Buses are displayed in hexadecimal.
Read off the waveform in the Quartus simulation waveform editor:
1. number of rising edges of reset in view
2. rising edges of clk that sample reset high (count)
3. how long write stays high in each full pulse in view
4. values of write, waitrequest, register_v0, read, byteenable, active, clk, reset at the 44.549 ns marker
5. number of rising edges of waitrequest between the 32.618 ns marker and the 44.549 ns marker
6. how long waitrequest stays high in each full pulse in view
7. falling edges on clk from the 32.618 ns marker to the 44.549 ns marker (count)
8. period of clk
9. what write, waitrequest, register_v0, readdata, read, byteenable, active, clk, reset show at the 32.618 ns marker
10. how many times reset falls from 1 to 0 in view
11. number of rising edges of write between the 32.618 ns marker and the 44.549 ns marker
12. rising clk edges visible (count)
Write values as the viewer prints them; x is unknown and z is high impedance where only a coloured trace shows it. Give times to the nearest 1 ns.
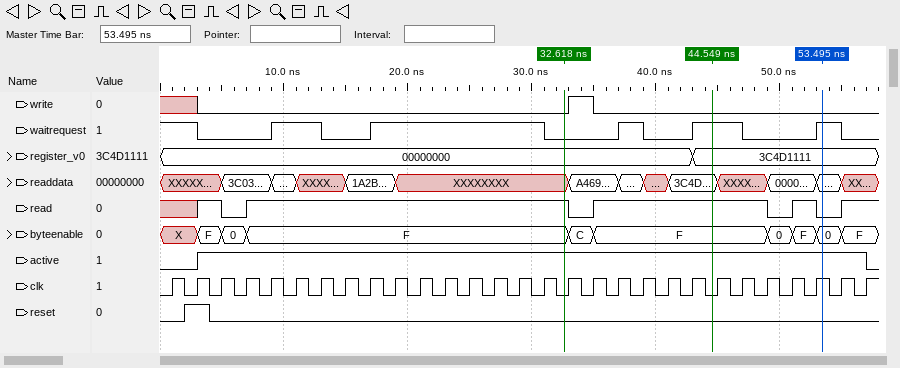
1
1
2 ns
write=0, waitrequest=1, register_v0=3C4D1111, read=1, byteenable=F, active=1, clk=0, reset=0
2
4 ns, 14 ns, 2 ns, 4 ns, 2 ns
6
2 ns
write=0, waitrequest=0, register_v0=00000000, readdata=XXXXXXXX, read=1, byteenable=F, active=1, clk=0, reset=0
1
1
29
